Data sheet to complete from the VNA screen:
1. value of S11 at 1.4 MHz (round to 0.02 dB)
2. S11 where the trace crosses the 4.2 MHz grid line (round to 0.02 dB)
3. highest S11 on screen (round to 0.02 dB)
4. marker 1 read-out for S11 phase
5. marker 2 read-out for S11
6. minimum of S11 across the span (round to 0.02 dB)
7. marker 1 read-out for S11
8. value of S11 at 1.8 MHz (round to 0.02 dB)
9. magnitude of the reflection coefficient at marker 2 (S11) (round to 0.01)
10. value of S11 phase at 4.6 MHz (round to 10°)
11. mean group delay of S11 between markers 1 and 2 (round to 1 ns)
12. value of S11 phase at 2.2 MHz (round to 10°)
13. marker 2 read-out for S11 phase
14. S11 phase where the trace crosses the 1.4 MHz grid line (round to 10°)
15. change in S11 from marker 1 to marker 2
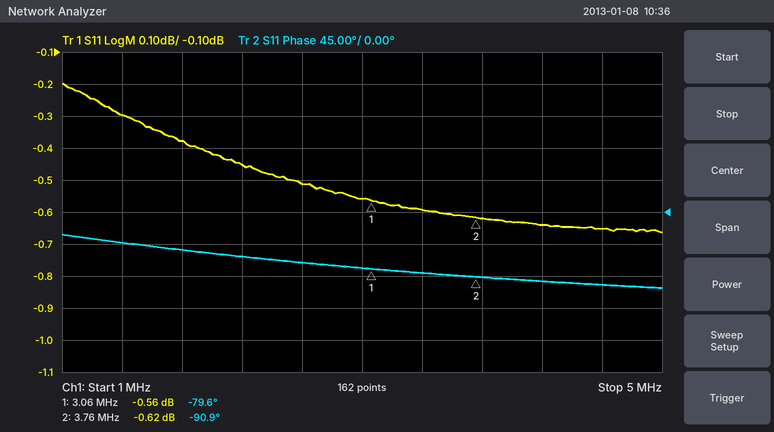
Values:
-0.30 dB
-0.64 dB
-0.20 dB
-79.6°
-0.62 dB
-0.66 dB
-0.56 dB
-0.38 dB
0.93
-100°
45 ns
-60°
-90.9°
-40°
-0.06 dB
